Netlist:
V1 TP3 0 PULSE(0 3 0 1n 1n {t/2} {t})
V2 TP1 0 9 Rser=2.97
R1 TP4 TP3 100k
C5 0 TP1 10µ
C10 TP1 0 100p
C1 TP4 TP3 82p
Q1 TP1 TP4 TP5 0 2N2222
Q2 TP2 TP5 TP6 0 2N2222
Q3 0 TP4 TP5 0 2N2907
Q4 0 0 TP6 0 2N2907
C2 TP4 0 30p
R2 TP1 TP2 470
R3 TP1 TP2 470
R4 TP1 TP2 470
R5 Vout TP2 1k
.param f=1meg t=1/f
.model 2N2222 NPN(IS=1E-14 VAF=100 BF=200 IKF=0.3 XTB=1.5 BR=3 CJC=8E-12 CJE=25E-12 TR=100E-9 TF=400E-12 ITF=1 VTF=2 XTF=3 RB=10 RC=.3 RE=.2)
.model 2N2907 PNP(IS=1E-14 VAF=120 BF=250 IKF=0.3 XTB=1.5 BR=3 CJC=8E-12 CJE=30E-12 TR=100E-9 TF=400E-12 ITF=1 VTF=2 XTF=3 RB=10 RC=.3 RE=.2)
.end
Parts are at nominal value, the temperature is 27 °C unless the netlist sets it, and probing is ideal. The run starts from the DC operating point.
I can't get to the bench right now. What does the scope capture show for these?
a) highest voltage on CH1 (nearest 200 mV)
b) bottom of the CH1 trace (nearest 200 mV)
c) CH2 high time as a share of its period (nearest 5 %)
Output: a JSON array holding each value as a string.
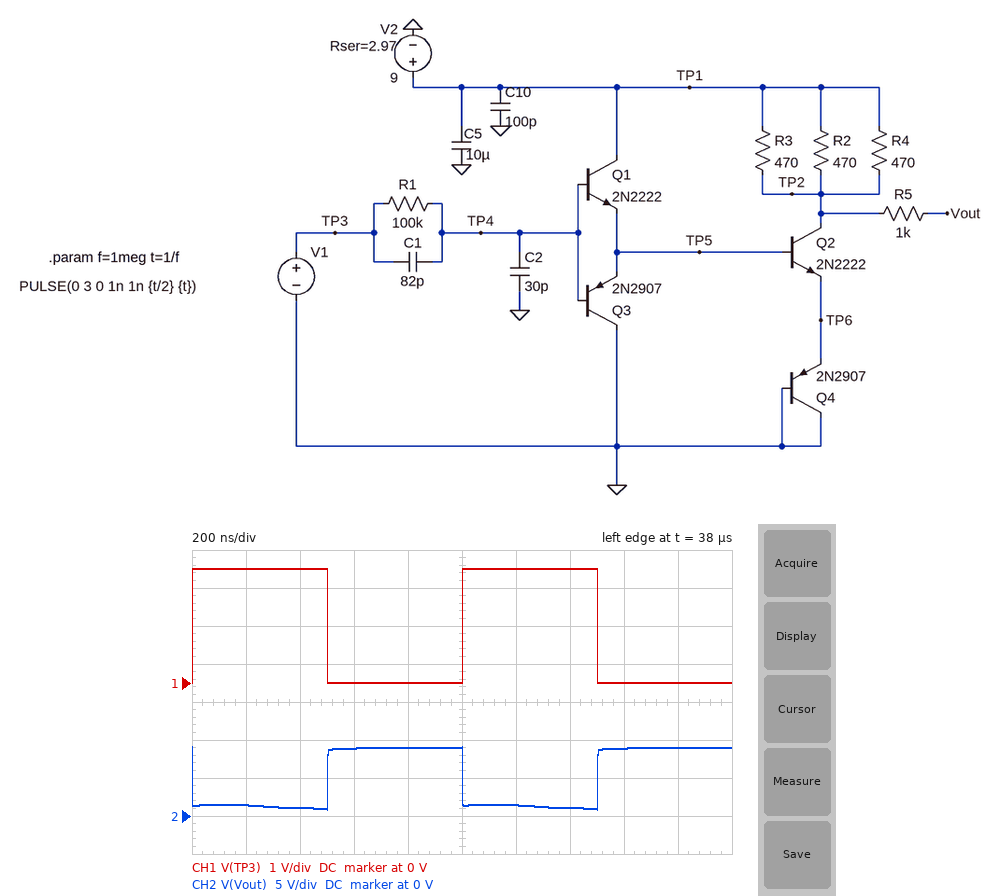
["3.0 V", "0 V", "50 %"]
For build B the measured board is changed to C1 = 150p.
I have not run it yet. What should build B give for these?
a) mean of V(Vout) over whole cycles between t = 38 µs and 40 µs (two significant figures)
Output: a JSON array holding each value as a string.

["4.8 V"]
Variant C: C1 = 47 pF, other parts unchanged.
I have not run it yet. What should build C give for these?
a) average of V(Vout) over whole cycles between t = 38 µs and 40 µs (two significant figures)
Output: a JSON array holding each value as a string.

["7.3 V"]
